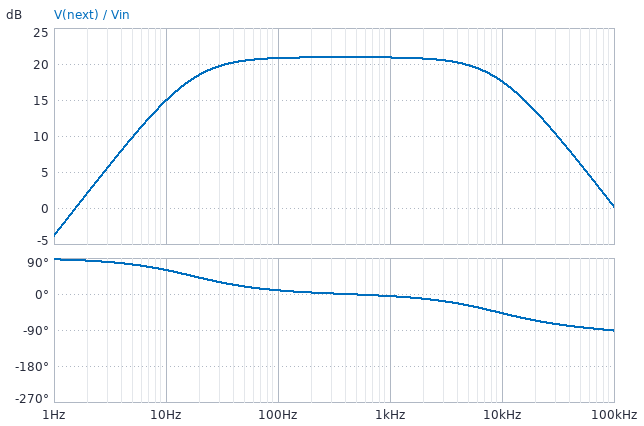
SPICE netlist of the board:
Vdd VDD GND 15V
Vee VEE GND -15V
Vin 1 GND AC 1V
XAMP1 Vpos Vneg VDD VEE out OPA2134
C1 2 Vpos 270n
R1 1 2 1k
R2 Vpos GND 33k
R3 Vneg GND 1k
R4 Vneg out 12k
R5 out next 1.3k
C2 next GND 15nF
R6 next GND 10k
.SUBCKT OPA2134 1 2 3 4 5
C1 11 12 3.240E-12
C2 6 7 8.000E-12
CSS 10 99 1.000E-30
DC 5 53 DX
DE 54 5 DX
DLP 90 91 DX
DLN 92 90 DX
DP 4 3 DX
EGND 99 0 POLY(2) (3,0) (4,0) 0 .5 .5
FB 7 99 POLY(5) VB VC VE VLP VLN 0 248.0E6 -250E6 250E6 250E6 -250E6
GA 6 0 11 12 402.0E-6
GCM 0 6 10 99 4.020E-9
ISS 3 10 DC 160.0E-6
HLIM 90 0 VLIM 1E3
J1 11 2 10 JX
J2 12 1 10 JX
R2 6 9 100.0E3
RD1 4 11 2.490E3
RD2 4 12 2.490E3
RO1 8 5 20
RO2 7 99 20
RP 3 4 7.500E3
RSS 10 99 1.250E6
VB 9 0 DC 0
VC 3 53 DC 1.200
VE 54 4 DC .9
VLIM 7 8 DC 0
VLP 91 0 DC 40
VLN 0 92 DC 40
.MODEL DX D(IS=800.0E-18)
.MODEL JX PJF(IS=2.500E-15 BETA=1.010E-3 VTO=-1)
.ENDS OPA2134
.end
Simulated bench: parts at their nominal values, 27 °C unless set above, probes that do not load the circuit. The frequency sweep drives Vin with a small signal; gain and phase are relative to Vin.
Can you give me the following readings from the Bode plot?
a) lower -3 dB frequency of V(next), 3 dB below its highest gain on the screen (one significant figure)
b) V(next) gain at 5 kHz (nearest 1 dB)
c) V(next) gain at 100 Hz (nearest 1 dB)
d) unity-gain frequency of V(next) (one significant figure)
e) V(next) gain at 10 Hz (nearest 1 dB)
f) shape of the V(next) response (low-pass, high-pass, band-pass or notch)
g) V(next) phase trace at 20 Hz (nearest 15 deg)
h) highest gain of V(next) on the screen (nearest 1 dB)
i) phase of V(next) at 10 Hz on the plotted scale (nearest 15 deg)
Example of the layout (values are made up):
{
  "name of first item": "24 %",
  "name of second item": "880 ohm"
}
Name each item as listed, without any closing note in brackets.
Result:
{
  "lower -3 dB frequency of V(next), 3 dB below its highest gain on the screen": "20 Hz",
  "V(next) gain at 5 kHz": "20 dB",
  "V(next) gain at 100 Hz": "21 dB",
  "unity-gain frequency of V(next)": "2 Hz",
  "V(next) gain at 10 Hz": "15 dB",
  "shape of the V(next) response": "band-pass",
  "V(next) phase trace at 20 Hz": "45 deg",
  "highest gain of V(next) on the screen": "21 dB",
  "phase of V(next) at 10 Hz on the plotted scale": "60 deg"
}
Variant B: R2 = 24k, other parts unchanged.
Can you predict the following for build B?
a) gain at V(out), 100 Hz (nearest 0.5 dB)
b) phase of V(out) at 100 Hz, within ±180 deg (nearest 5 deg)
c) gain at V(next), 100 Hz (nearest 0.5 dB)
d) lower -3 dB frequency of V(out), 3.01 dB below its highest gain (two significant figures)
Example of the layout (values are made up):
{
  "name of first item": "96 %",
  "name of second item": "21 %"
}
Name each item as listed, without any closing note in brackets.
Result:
{
  "gain at V(out), 100 Hz": "21.5 dB",
  "phase of V(out) at 100 Hz, within ±180 deg": "15 deg",
  "gain at V(next), 100 Hz": "20.5 dB",
  "lower -3 dB frequency of V(out), 3.01 dB below its highest gain": "24 Hz"
}
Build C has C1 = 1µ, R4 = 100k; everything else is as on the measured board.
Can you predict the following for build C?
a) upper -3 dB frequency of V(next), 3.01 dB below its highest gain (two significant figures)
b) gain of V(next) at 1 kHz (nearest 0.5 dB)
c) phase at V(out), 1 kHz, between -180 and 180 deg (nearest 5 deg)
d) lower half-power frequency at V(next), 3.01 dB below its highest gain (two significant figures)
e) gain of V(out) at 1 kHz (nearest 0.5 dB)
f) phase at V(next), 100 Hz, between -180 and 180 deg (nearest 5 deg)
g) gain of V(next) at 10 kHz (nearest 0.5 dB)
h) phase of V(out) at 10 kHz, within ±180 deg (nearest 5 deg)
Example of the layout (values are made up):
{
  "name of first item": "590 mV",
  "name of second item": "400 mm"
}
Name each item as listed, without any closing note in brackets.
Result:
{
  "upper -3 dB frequency of V(next), 3.01 dB below its highest gain": "9.2 kHz",
  "gain of V(next) at 1 kHz": "38.5 dB",
  "phase at V(out), 1 kHz, between -180 and 180 deg": "0 deg",
  "lower half-power frequency at V(next), 3.01 dB below its highest gain": "4.7 Hz",
  "gain of V(out) at 1 kHz": "40.0 dB",
  "phase at V(next), 100 Hz, between -180 and 180 deg": "0 deg",
  "gain of V(next) at 10 kHz": "35.5 dB",
  "phase of V(out) at 10 kHz, within ±180 deg": "-5 deg"
}
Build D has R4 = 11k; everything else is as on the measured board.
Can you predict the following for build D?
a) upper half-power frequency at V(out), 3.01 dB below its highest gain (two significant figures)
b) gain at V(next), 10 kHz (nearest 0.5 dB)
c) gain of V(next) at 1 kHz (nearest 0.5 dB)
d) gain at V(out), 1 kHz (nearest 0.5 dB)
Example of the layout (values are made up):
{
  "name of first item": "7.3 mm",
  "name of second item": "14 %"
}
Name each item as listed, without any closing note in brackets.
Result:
{
  "upper half-power frequency at V(out), 3.01 dB below its highest gain": "1.0 MHz",
  "gain at V(next), 10 kHz": "17.0 dB",
  "gain of V(next) at 1 kHz": "20.0 dB",
  "gain at V(out), 1 kHz": "21.5 dB"
}
